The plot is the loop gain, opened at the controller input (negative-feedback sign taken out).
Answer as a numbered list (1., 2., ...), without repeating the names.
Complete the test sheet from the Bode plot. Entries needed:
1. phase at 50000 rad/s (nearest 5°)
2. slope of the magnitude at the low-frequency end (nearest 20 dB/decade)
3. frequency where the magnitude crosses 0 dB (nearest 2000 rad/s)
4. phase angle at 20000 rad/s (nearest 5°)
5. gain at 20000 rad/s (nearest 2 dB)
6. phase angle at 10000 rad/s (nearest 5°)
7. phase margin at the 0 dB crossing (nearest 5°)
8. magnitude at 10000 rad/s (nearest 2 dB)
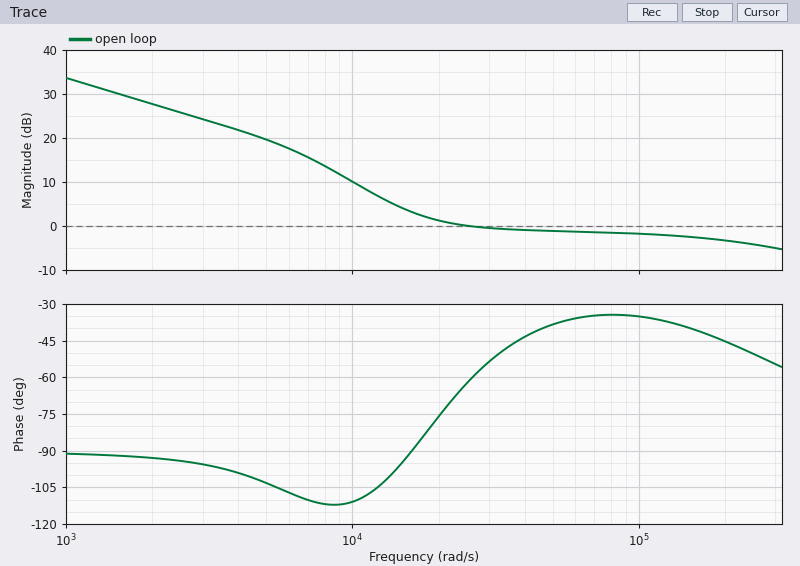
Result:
1. -40°
2. -20 dB/decade
3. 26000 rad/s
4. -75°
5. 2 dB
6. -110°
7. 120°
8. 10 dB
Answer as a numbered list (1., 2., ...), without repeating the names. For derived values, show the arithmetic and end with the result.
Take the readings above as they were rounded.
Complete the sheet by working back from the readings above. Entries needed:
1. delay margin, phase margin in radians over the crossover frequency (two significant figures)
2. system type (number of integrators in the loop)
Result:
1. 120 × π / 180 / 26000 = 0.000081 s
2. 1
